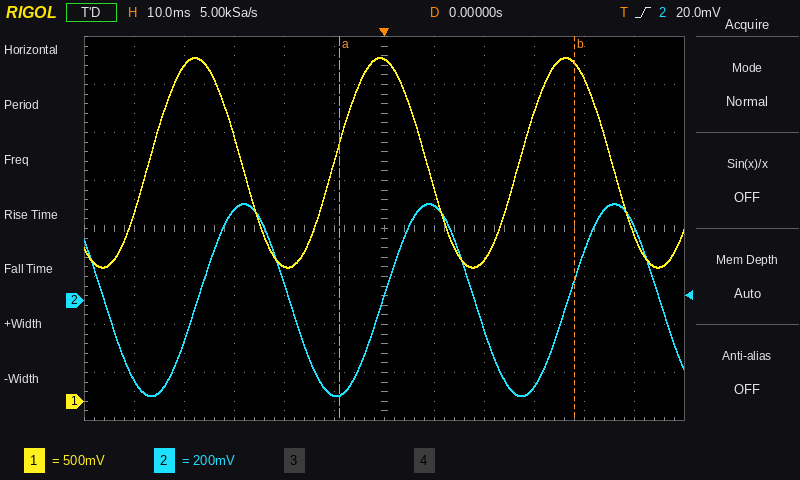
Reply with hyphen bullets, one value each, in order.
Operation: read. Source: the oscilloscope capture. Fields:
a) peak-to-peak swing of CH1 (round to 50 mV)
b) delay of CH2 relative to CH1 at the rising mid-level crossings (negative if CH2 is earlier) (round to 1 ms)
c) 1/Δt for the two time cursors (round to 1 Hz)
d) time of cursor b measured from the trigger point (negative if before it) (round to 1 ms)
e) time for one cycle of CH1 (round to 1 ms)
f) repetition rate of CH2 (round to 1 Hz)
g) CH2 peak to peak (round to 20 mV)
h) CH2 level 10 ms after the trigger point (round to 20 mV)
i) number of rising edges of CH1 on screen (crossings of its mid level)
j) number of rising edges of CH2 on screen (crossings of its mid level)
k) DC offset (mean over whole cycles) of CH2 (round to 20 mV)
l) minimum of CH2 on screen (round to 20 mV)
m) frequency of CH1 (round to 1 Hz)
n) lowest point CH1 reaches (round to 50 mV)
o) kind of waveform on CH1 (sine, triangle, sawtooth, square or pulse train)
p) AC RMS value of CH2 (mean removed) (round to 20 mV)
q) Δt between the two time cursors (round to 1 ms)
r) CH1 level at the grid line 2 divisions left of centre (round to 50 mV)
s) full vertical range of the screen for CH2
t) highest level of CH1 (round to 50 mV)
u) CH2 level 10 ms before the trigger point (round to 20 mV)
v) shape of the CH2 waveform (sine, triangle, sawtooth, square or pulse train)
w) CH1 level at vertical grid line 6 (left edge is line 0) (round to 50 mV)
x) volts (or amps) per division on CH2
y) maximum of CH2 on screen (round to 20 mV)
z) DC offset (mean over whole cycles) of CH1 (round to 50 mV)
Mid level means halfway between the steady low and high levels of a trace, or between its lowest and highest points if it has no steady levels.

- 2.20 V
- +10 ms
- 21 Hz
- +38 ms
- 37 ms
- 27 Hz
- 800 mV
- 400 mV
- 3
- 3
- 0 mV
- -400 mV
- 27 Hz
- 1.40 V
- sine
- 280 mV
- 47 ms
- 1.40 V
- 1.6 V
- 3.60 V
- -400 mV
- sine
- 3.55 V
- 200 mV
- 400 mV
- 2.50 V
